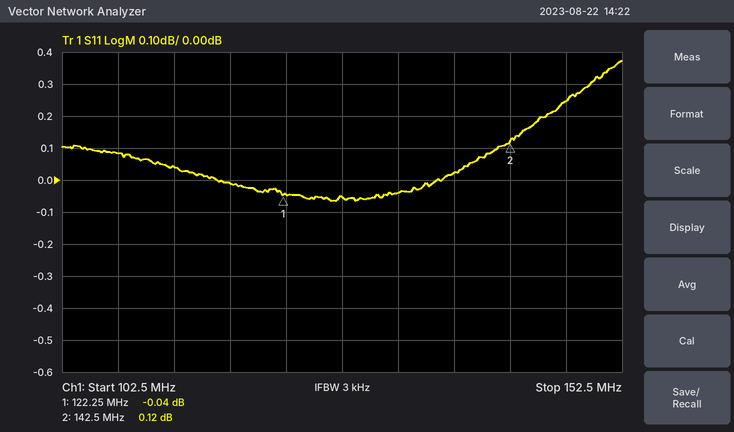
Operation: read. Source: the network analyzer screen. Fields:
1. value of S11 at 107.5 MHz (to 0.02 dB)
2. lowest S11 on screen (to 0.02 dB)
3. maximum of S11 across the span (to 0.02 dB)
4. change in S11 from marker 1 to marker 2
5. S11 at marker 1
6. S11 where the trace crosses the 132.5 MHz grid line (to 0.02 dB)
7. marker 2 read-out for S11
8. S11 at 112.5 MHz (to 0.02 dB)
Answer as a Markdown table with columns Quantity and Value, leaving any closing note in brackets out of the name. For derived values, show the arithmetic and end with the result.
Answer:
| Quantity | Value |
|---|---|
| value of S11 at 107.5 MHz | 0.08 dB |
| lowest S11 on screen | -0.06 dB |
| maximum of S11 across the span | 0.38 dB |
| change in S11 from marker 1 to marker 2 | 0.12 − (-0.04) = 0.16 dB |
| S11 at marker 1 | -0.04 dB |
| S11 where the trace crosses the 132.5 MHz grid line | -0.04 dB |
| marker 2 read-out for S11 | 0.12 dB |
| S11 at 112.5 MHz | 0.04 dB |
